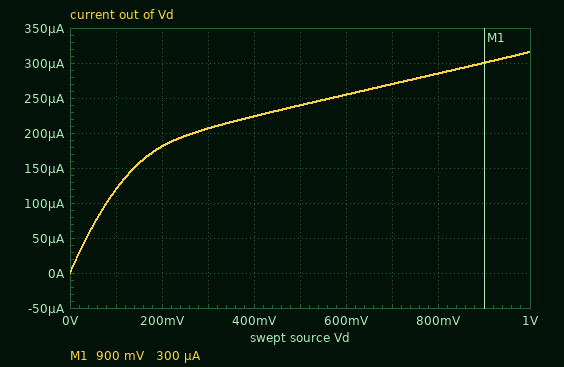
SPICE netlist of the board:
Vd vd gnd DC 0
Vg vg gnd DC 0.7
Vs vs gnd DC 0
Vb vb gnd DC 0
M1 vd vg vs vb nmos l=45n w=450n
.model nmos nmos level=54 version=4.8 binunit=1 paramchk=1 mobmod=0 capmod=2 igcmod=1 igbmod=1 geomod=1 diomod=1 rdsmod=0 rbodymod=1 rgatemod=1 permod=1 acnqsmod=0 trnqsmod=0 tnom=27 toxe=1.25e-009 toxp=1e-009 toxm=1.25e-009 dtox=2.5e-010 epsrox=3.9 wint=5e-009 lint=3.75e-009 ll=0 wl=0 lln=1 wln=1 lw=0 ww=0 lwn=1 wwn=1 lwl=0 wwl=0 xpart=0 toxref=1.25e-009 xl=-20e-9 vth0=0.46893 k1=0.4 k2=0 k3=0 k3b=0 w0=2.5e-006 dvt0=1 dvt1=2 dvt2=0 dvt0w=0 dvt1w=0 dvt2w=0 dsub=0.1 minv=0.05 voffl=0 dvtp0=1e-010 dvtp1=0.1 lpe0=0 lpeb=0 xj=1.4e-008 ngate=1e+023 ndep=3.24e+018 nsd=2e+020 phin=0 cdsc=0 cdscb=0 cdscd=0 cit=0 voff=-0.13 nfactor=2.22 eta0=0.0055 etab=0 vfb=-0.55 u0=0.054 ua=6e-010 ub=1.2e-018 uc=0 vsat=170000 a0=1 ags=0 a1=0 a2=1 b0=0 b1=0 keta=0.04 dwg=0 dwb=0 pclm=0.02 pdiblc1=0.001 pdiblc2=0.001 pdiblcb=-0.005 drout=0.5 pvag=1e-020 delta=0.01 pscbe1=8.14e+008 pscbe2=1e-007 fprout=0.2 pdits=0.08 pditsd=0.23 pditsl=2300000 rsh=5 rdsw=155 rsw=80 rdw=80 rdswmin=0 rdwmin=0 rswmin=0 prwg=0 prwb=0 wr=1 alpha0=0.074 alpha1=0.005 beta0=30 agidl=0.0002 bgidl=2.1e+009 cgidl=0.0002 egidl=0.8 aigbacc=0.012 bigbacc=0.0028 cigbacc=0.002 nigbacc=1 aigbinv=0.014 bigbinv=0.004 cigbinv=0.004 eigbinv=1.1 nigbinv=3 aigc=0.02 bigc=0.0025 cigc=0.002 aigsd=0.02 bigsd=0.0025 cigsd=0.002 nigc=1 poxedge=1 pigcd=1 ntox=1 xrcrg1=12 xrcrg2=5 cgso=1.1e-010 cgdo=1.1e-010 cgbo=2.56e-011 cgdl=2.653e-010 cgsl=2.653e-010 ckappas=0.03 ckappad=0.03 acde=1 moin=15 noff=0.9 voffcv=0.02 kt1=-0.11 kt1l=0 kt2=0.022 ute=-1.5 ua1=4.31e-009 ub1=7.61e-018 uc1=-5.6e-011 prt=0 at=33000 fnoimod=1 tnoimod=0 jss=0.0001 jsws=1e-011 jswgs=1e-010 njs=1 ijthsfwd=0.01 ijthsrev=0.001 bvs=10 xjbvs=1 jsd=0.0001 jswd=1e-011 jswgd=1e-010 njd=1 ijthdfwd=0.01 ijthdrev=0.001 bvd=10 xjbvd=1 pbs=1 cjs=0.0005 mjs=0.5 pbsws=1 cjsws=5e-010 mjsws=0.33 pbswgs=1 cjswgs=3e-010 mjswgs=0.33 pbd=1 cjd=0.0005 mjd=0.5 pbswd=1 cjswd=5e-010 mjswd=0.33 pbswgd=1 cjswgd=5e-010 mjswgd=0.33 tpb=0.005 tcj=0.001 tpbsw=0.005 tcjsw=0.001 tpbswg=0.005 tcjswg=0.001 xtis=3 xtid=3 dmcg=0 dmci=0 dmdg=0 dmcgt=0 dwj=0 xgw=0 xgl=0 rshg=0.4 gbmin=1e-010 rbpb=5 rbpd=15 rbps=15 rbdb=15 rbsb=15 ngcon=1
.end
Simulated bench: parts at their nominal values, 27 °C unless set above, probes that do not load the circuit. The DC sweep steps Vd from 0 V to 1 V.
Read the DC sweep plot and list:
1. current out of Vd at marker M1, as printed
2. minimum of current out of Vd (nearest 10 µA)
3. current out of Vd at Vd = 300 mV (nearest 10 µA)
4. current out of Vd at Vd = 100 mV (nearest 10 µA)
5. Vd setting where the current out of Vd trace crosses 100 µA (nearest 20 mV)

300 µA
0 A
210 µA
120 µA
80 mV
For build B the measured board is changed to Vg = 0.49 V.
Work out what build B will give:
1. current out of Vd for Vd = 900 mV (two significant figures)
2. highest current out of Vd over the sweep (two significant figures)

110 µA
120 µA
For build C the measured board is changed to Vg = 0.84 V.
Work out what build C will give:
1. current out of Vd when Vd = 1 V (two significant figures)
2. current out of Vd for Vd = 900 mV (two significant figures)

450 µA
430 µA
